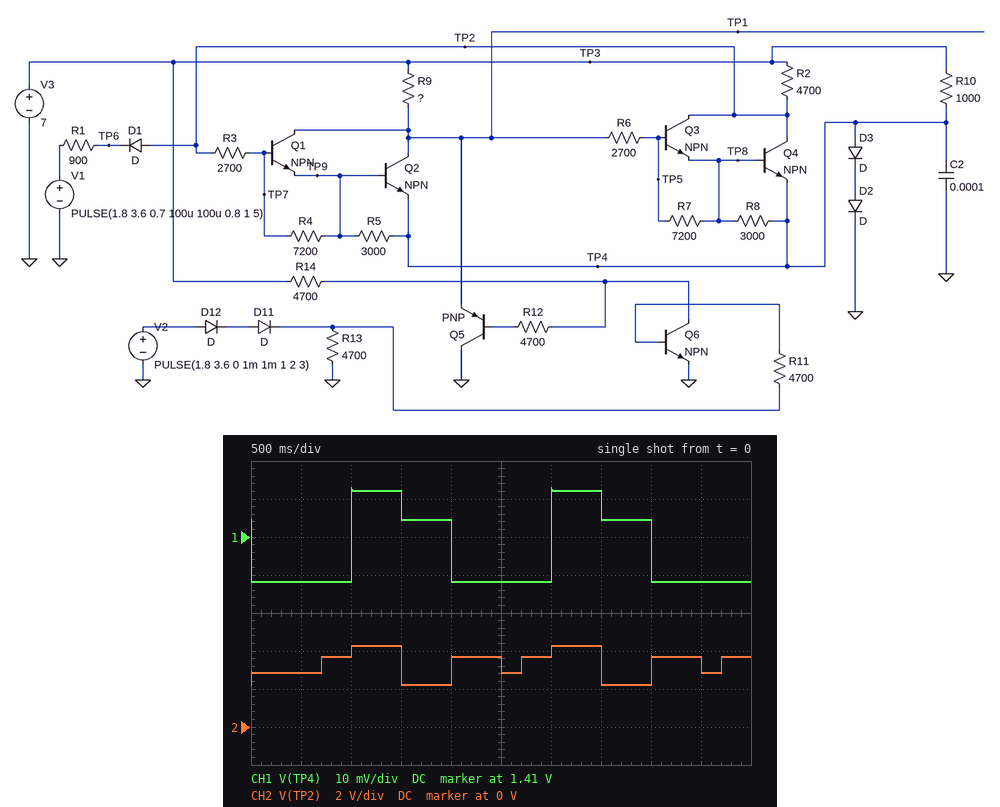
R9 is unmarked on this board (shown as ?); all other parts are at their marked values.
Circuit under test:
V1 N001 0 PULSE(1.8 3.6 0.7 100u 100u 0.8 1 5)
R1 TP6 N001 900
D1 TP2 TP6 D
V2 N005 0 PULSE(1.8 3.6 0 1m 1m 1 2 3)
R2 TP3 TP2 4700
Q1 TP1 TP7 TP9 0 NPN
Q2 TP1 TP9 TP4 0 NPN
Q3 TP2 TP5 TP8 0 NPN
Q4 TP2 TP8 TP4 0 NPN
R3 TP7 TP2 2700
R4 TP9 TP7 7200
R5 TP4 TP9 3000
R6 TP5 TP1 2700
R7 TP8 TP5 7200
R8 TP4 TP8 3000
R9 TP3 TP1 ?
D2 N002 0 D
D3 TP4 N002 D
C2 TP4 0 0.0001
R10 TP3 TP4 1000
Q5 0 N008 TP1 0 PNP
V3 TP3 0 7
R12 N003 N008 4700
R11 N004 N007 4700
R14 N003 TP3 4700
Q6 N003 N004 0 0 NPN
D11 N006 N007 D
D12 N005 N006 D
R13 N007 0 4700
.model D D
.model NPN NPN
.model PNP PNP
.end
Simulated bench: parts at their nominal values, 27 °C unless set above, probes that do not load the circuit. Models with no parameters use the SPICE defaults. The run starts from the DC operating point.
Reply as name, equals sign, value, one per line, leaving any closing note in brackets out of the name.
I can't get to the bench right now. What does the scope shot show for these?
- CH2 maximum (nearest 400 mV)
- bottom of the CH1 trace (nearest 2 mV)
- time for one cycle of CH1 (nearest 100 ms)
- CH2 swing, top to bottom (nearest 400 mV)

CH2 maximum = 4.4 V
bottom of the CH1 trace = 1.398 V
time for one cycle of CH1 = 2.0 s
CH2 swing, top to bottom = 2.0 V
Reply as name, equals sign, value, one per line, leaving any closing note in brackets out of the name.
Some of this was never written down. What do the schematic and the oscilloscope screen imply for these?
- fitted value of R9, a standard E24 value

fitted value of R9, a standard E24 value = 1.8 kΩ
